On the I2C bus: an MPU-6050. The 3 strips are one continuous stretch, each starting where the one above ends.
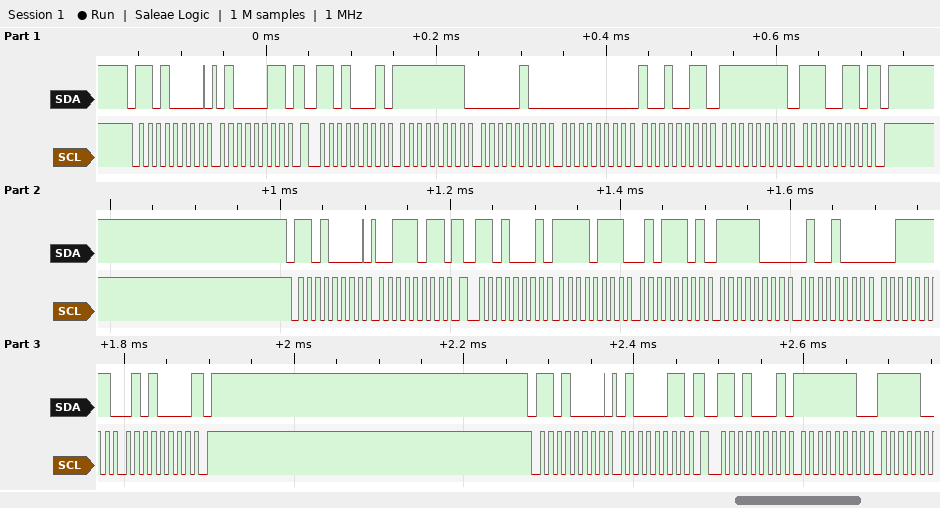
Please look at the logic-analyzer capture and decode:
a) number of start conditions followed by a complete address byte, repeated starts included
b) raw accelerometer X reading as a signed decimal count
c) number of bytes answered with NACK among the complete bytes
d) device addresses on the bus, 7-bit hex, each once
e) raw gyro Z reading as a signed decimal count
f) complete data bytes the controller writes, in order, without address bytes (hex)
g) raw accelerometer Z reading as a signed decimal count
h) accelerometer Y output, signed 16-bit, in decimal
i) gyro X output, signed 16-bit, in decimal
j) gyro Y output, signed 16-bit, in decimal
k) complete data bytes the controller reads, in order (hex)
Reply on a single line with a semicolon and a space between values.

6; -2211; 2; 0x68; -26; 43 3B 43; 16208; -1976; -252; 147; FF 04 00 93 FF E6 F7 5D F8 48 3F 50 FE
